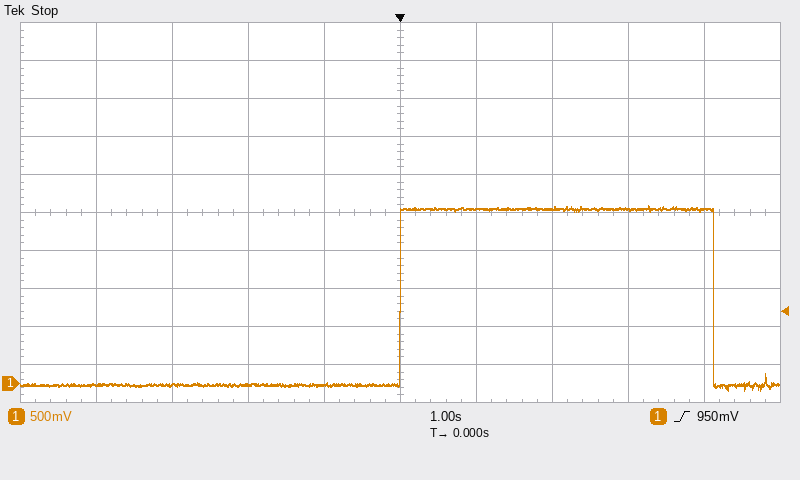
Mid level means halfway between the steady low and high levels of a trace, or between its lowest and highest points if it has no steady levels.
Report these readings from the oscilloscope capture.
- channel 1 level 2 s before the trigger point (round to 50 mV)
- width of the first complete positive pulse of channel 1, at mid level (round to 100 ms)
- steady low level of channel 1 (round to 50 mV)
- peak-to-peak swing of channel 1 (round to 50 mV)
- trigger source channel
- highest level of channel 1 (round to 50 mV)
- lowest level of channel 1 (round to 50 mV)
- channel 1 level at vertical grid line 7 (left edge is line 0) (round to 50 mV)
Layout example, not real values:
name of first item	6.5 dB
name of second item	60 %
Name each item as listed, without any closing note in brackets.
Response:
channel 1 level 2 s before the trigger point	0 mV
width of the first complete positive pulse of channel 1, at mid level	4.1 s
steady low level of channel 1	0 mV
peak-to-peak swing of channel 1	2.45 V
trigger source channel	channel 1
highest level of channel 1	2.35 V
lowest level of channel 1	-100 mV
channel 1 level at vertical grid line 7 (left edge is line 0)	2.30 V
